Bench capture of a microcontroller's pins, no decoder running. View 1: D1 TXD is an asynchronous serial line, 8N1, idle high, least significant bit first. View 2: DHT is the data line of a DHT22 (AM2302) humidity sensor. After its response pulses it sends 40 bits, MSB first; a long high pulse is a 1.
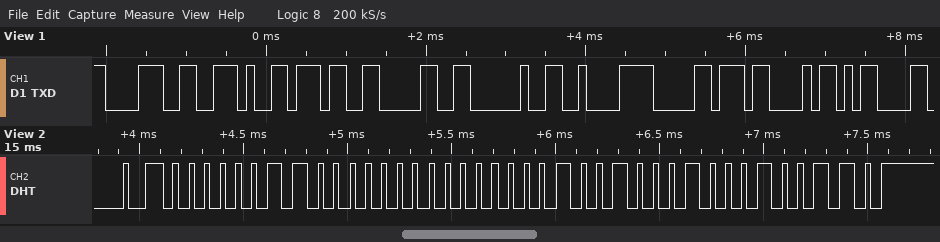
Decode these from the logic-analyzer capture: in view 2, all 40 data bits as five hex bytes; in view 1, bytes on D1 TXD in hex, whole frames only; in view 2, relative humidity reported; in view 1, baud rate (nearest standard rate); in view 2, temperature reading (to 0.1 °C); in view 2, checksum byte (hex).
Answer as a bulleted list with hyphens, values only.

- 03 00 01 22 26
- 38 2E 37 30 20 C2 B0 43 0D
- 76.8 %
- 9600 baud
- 29.0 °C
- 0x26
